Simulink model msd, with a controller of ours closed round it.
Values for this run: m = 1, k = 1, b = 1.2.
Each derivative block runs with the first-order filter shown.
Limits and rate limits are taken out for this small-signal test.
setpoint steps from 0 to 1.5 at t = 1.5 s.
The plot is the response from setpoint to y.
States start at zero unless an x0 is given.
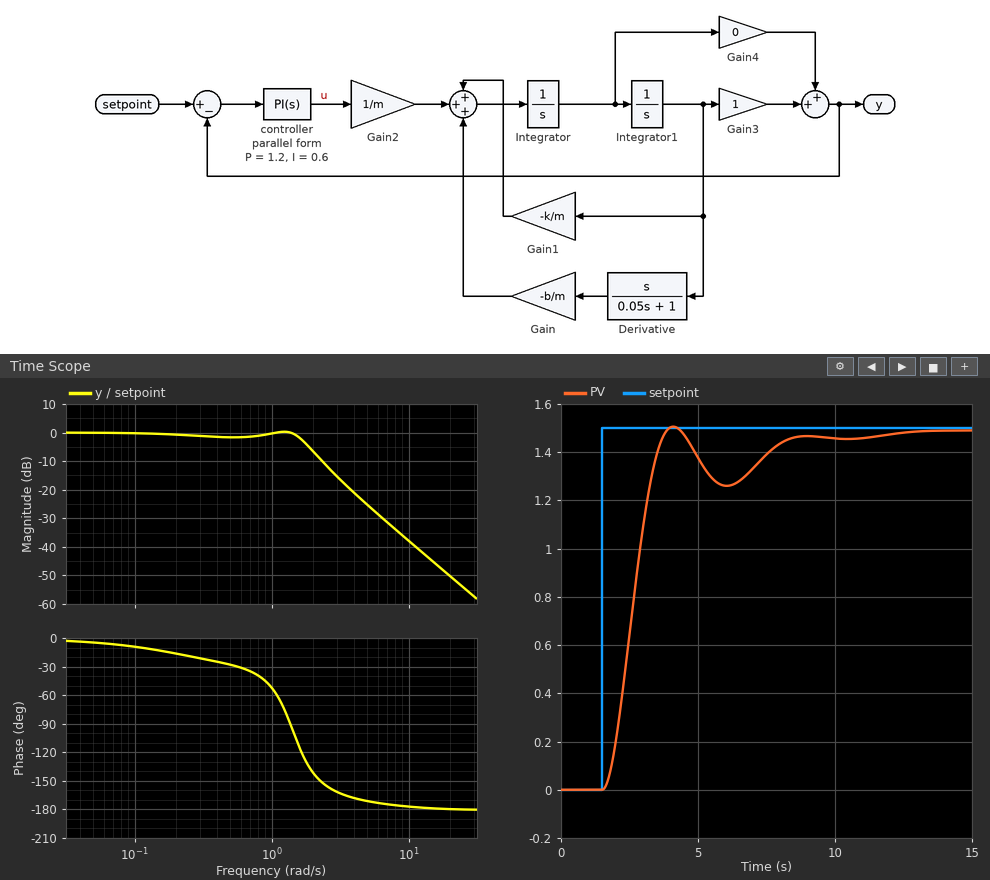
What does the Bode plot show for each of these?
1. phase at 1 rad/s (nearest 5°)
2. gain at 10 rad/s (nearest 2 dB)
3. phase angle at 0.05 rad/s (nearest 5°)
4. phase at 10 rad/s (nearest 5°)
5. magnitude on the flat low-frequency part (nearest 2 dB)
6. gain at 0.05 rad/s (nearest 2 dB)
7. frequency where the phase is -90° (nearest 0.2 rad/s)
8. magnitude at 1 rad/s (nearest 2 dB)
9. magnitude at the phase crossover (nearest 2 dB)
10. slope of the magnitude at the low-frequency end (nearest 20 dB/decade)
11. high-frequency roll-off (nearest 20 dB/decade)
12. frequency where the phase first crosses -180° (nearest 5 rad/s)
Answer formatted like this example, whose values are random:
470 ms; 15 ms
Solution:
-50°; -38 dB; -5°; -175°; 0 dB; 0 dB; 1.4 rad/s; 0 dB; -54 dB; 0 dB/decade; -40 dB/decade; 25 rad/s
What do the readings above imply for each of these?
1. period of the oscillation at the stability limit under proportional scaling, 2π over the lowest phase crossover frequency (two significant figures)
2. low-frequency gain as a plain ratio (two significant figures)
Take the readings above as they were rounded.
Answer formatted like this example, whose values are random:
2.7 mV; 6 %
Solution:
0.25 s; 1.0
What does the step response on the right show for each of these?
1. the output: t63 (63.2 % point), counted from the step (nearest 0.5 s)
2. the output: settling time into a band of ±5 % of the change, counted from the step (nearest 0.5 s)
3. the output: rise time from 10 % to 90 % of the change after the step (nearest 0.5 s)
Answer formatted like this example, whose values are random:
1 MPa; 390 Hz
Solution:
1.5 s; 6.5 s; 1.5 s
